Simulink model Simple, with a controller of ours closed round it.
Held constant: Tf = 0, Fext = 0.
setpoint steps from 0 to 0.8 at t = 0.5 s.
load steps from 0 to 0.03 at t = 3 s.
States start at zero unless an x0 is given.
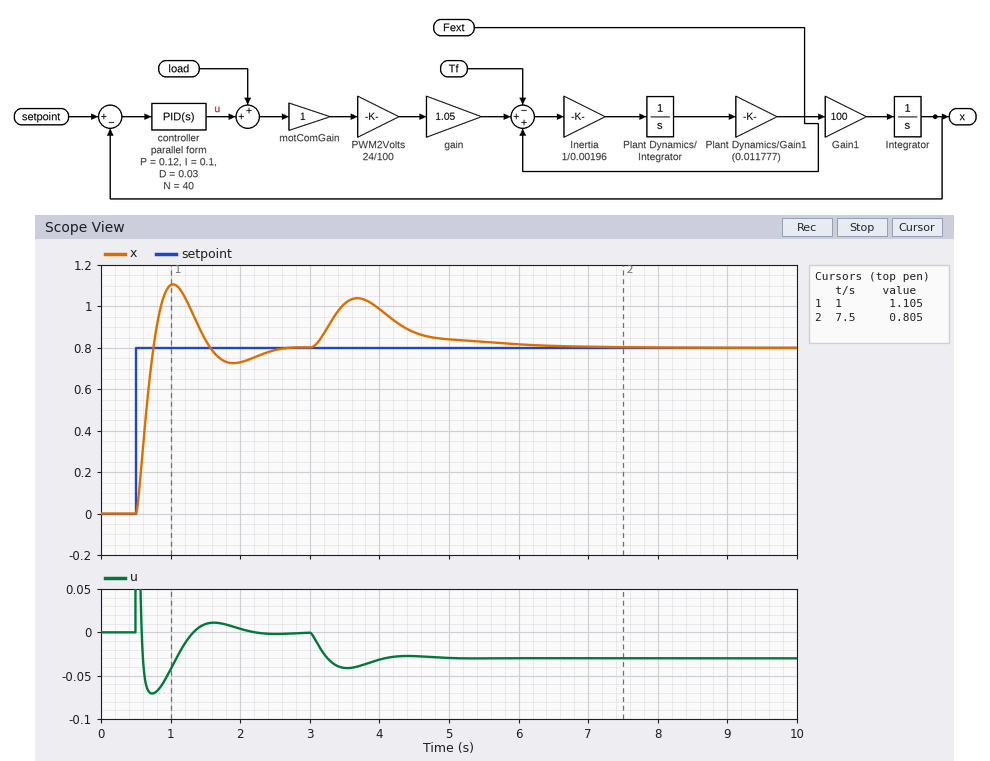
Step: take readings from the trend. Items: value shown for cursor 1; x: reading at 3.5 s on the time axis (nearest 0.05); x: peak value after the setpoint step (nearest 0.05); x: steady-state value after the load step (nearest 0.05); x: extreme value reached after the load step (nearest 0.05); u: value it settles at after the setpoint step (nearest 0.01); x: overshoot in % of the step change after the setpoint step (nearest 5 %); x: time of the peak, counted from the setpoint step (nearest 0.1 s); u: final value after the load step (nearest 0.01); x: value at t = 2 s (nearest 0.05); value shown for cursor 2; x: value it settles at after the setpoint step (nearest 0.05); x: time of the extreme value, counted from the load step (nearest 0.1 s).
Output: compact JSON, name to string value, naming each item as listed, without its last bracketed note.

{"value shown for cursor 1": "1.105", "x: reading at 3.5 s on the time axis": "1.00", "x: peak value after the setpoint step": "1.10", "x: steady-state value after the load step": "0.80", "x: extreme value reached after the load step": "1.05", "u: value it settles at after the setpoint step": "0.00", "x: overshoot in % of the step change after the setpoint step": "40 %", "x: time of the peak, counted from the setpoint step": "0.5 s", "u: final value after the load step": "-0.03", "x: value at t = 2 s": "0.75", "value shown for cursor 2": "0.805", "x: value it settles at after the setpoint step": "0.80", "x: time of the extreme value, counted from the load step": "0.7 s"}
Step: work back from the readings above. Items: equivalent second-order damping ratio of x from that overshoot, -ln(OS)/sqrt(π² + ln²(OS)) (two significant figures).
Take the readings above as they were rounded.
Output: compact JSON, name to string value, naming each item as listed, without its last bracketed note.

{"equivalent second-order damping ratio of x from that overshoot, -ln(OS)/sqrt(π² + ln²(OS))": "0.28"}
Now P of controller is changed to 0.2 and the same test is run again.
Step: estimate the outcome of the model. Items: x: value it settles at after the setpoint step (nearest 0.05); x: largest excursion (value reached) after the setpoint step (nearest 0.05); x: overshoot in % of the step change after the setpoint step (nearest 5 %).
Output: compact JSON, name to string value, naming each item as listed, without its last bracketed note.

{"x: value it settles at after the setpoint step": "0.80", "x: largest excursion (value reached) after the setpoint step": "1.15", "x: overshoot in % of the step change after the setpoint step": "45 %"}
